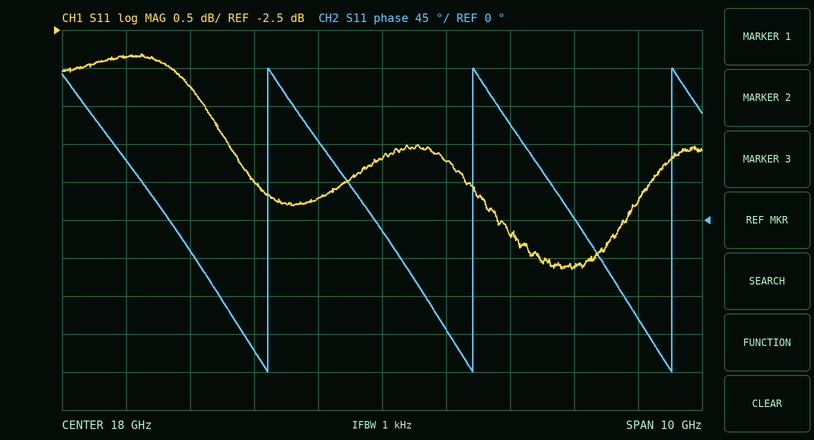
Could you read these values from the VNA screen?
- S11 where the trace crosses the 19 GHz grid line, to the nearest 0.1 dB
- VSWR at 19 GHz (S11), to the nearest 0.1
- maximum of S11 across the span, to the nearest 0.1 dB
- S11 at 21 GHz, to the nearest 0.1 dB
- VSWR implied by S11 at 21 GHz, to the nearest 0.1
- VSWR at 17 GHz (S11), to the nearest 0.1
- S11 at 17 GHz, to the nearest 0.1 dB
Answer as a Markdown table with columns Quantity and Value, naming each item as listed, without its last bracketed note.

| Quantity | Value |
|---|---|
| S11 where the trace crosses the 19 GHz grid line, to the nearest 0.1 dB | -4.2 dB |
| VSWR at 19 GHz (S11), to the nearest 0.1 | 4.2 |
| maximum of S11 across the span, to the nearest 0.1 dB | -2.8 dB |
| S11 at 21 GHz, to the nearest 0.1 dB | -5.6 dB |
| VSWR implied by S11 at 21 GHz, to the nearest 0.1 | 3.2 |
| VSWR at 17 GHz (S11), to the nearest 0.1 | 3.8 |
| S11 at 17 GHz, to the nearest 0.1 dB | -4.7 dB |
